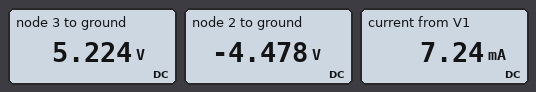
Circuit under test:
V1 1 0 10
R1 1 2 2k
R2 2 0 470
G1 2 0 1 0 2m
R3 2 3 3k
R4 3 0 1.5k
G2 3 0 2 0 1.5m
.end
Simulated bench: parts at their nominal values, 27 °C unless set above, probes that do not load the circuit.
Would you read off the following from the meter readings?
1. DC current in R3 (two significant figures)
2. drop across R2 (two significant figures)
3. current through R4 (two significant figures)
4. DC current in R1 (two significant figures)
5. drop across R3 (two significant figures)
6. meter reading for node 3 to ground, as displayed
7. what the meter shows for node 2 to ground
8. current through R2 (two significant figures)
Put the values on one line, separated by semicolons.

3.2 mA; 4.5 V; 3.5 mA; 7.2 mA; 9.7 V; 5.224 V; -4.478 V; 9.5 mA
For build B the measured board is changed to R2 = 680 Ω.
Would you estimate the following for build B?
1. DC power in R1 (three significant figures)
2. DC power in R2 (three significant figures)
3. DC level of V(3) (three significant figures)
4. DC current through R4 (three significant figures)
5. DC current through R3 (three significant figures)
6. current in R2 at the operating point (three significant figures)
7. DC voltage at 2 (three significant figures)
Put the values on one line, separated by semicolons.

121 mW; 45.6 mW; 6.50 V; 4.33 mA; 4.02 mA; 8.19 mA; -5.57 V
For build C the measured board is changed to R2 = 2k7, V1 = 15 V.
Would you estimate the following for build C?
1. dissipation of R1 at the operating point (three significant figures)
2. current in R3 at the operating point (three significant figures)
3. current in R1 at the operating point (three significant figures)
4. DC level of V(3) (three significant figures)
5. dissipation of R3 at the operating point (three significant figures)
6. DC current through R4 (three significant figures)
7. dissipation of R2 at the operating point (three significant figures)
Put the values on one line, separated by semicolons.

424 mW; 10.2 mA; 14.6 mA; 16.5 V; 312 mW; 11.0 mA; 73.9 mW
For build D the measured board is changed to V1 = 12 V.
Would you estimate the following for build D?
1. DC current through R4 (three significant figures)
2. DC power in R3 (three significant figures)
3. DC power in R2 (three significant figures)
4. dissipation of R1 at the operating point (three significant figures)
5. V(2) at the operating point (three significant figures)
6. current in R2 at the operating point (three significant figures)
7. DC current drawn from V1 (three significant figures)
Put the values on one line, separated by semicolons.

4.18 mA; 45.2 mW; 61.4 mW; 151 mW; -5.37 V; 11.4 mA; 8.69 mA
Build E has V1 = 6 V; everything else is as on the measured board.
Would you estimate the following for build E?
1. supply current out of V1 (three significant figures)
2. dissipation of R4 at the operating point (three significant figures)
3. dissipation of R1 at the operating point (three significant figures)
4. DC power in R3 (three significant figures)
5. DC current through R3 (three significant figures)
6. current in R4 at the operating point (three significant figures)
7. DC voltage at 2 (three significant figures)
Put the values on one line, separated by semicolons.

4.34 mA; 6.55 mW; 37.7 mW; 11.3 mW; 1.94 mA; 2.09 mA; -2.69 V
